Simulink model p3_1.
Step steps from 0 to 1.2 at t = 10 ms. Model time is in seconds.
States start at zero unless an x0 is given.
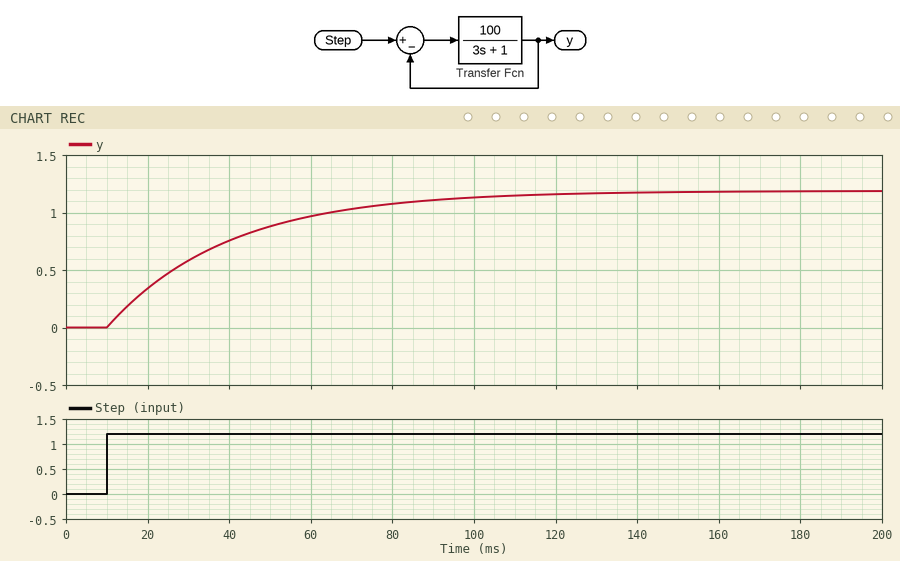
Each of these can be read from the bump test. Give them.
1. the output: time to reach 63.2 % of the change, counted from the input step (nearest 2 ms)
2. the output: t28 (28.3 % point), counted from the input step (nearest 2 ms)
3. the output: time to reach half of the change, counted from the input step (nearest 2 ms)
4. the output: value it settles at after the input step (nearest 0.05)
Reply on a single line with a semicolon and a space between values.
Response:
30 ms; 10 ms; 20 ms; 1.20
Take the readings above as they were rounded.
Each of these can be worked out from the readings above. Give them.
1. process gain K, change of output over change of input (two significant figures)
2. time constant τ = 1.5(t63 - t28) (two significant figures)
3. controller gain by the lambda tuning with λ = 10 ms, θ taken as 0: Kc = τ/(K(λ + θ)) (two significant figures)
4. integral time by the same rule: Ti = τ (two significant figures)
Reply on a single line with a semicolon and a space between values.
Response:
1.0; 30 ms; 3.0; 30 ms
